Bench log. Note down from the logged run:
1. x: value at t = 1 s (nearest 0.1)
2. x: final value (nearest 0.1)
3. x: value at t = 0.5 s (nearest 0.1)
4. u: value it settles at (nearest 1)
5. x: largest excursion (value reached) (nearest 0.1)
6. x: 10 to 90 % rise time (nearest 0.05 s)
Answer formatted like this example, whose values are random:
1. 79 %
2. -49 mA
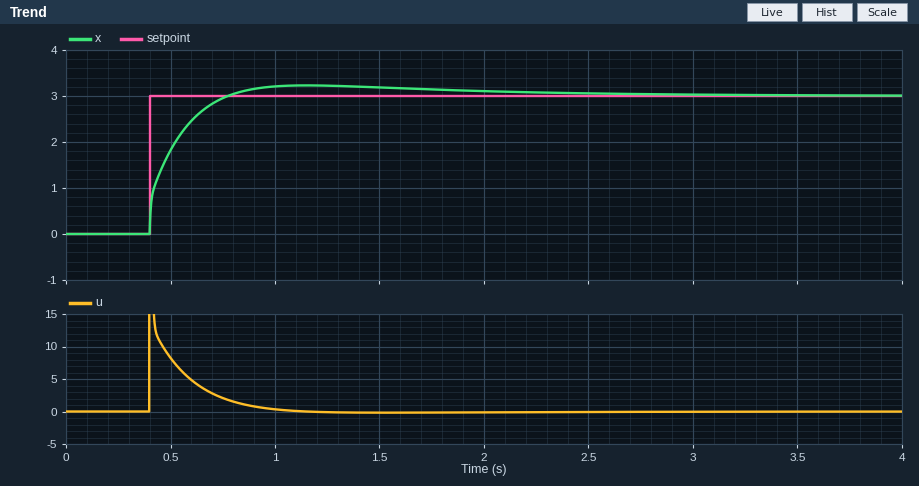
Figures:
1. 3.2
2. 3.0
3. 1.8
4. 0
5. 3.2
6. 0.25 s
